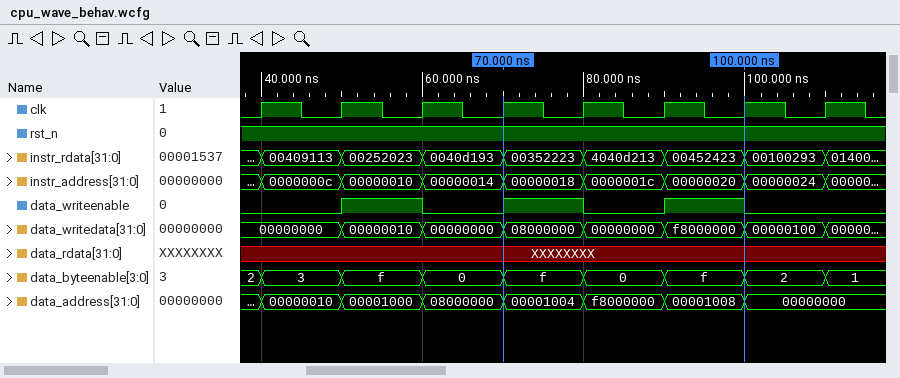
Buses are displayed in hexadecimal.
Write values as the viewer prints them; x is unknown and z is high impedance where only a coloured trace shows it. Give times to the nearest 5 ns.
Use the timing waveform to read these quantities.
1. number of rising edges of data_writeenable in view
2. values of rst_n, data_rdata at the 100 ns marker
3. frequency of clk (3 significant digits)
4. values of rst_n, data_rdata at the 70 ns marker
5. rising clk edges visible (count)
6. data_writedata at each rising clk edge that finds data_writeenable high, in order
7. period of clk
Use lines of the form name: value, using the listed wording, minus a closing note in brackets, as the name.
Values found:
number of rising edges of data_writeenable in view: 3
values of rst_n, data_rdata at the 100 ns marker: rst_n=1, data_rdata=XXXXXXXX
frequency of clk: 100 MHz
values of rst_n, data_rdata at the 70 ns marker: rst_n=1, data_rdata=XXXXXXXX
rising clk edges visible: 8
data_writedata at each rising clk edge that finds data_writeenable high, in order: 00000010, 08000000, f8000000
period of clk: 10 ns
